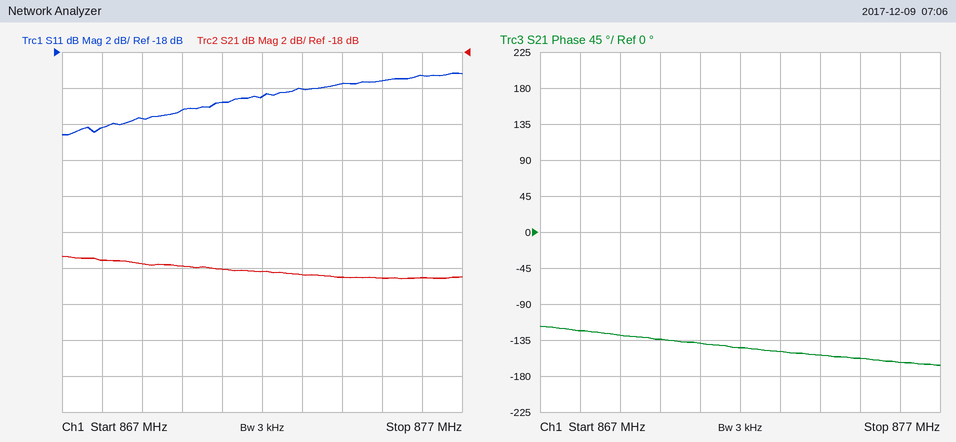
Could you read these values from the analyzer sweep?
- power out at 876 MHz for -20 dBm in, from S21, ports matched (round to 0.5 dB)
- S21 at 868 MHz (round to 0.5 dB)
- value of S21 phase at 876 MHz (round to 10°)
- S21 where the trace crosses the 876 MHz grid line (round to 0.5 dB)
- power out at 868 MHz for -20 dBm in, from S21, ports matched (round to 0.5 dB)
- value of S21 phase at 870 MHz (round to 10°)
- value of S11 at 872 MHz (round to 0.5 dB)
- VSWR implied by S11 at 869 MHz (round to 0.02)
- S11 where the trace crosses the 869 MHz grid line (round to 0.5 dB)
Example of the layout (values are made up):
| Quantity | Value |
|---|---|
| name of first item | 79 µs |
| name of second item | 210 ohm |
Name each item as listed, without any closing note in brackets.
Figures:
| Quantity | Value |
|---|---|
| power out at 876 MHz for -20 dBm in, from S21, ports matched | -50.5 dBm |
| S21 at 868 MHz | -29.5 dB |
| value of S21 phase at 876 MHz | -160° |
| S21 where the trace crosses the 876 MHz grid line | -30.5 dB |
| power out at 868 MHz for -20 dBm in, from S21, ports matched | -49.5 dBm |
| value of S21 phase at 870 MHz | -130° |
| value of S11 at 872 MHz | -20.5 dB |
| VSWR implied by S11 at 869 MHz | 1.18 |
| S11 where the trace crosses the 869 MHz grid line | -21.5 dB |
